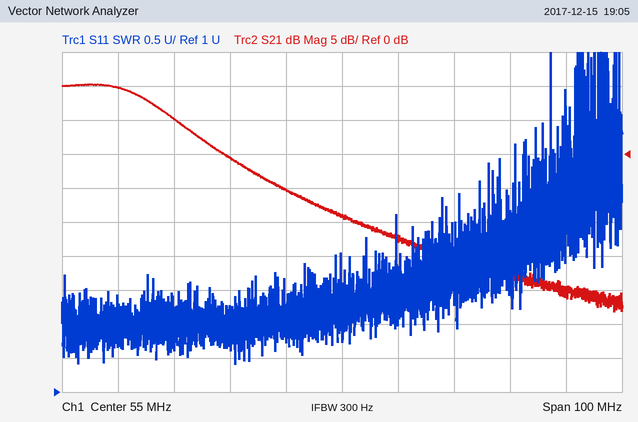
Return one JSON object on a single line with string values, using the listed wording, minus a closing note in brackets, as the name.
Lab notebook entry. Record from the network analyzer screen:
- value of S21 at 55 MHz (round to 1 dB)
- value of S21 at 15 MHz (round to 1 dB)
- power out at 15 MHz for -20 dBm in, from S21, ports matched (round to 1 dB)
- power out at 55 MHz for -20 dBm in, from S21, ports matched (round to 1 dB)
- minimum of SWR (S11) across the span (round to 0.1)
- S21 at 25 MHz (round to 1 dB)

{"value of S21 at 55 MHz": "-9 dB", "value of S21 at 15 MHz": "10 dB", "power out at 15 MHz for -20 dBm in, from S21, ports matched": "-10 dBm", "power out at 55 MHz for -20 dBm in, from S21, ports matched": "-29 dBm", "minimum of SWR (S11) across the span": "1.4", "S21 at 25 MHz": "5 dB"}
